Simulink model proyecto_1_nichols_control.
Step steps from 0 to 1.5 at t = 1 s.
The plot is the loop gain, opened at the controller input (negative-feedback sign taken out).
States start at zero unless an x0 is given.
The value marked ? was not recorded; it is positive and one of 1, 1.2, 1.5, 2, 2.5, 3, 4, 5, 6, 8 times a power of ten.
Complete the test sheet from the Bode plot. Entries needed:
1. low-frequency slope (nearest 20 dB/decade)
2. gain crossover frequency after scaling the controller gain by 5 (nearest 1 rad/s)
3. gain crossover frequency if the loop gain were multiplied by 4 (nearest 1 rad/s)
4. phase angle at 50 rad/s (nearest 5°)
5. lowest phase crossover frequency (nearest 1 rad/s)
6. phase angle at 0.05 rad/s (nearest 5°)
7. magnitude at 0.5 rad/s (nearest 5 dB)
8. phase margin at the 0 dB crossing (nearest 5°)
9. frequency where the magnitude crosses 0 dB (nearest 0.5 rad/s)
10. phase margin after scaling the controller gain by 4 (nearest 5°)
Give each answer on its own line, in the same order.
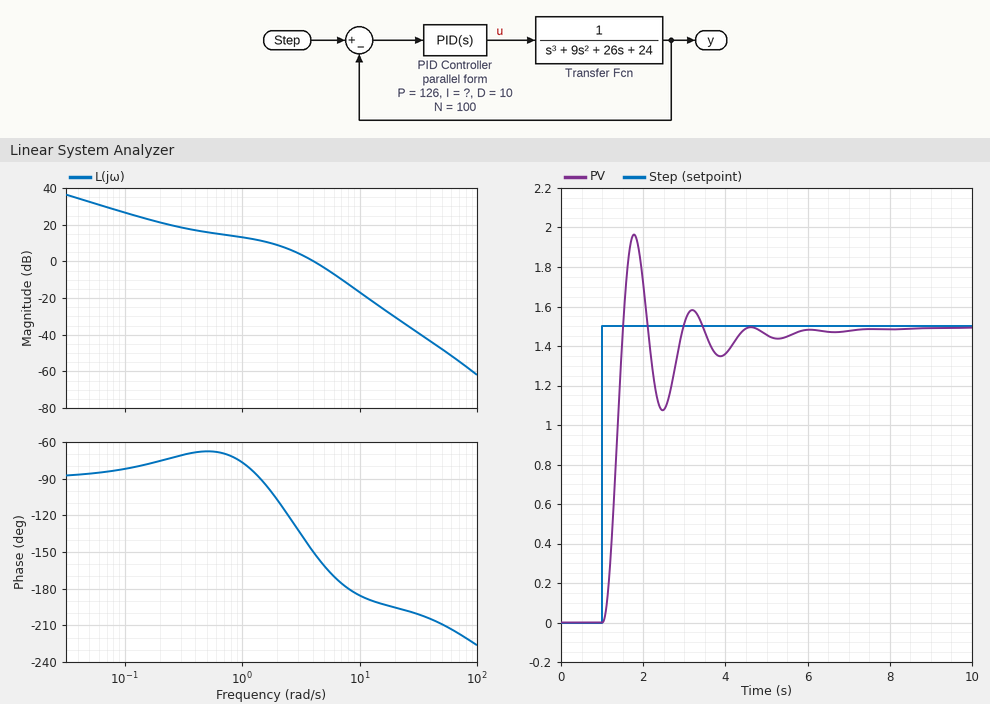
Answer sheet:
-20 dB/decade
9 rad/s
8 rad/s
-210°
8 rad/s
-85°
15 dB
30°
4.0 rad/s
0°
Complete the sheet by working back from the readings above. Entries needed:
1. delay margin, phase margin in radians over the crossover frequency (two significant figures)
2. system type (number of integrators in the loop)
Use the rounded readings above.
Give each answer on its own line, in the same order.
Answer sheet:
0.13 s
1
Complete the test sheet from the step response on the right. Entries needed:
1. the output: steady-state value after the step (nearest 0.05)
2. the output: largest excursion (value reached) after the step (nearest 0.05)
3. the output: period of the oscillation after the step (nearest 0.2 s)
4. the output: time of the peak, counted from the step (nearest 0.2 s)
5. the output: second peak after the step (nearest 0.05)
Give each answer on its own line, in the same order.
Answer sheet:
1.50
1.95
1.4 s
0.8 s
1.60
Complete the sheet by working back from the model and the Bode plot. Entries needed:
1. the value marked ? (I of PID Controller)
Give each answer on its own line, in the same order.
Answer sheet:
50
